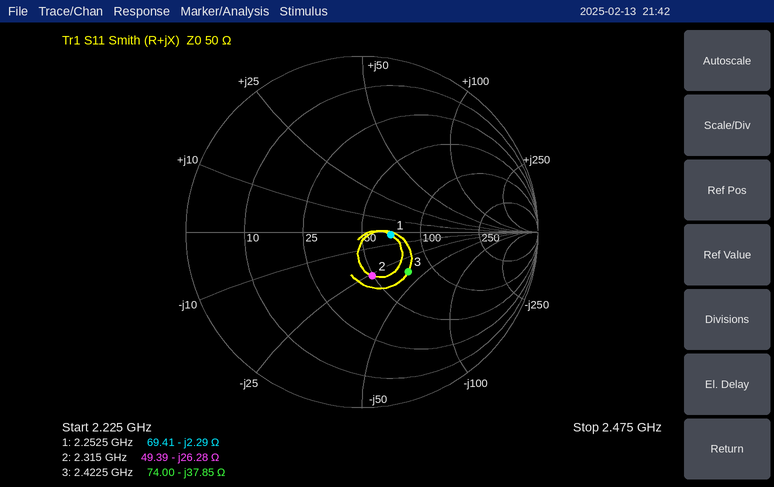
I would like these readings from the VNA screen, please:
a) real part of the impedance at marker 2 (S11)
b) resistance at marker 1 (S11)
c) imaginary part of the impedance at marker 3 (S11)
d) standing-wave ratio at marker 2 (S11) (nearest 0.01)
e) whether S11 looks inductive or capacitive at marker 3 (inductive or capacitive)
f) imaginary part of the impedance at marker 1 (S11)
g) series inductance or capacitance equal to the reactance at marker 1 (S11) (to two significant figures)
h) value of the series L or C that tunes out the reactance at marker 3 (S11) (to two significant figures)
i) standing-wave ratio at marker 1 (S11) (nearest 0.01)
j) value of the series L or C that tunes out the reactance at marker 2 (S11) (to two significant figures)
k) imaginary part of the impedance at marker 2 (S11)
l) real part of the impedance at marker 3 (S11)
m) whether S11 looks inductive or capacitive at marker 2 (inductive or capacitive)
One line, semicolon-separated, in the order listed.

49.39 Ω; 69.41 Ω; -37.85 Ω; 1.69; capacitive; -2.29 Ω; 31 pF; 2.5 nH; 1.39; 1.8 nH; -26.28 Ω; 74.00 Ω; capacitive
